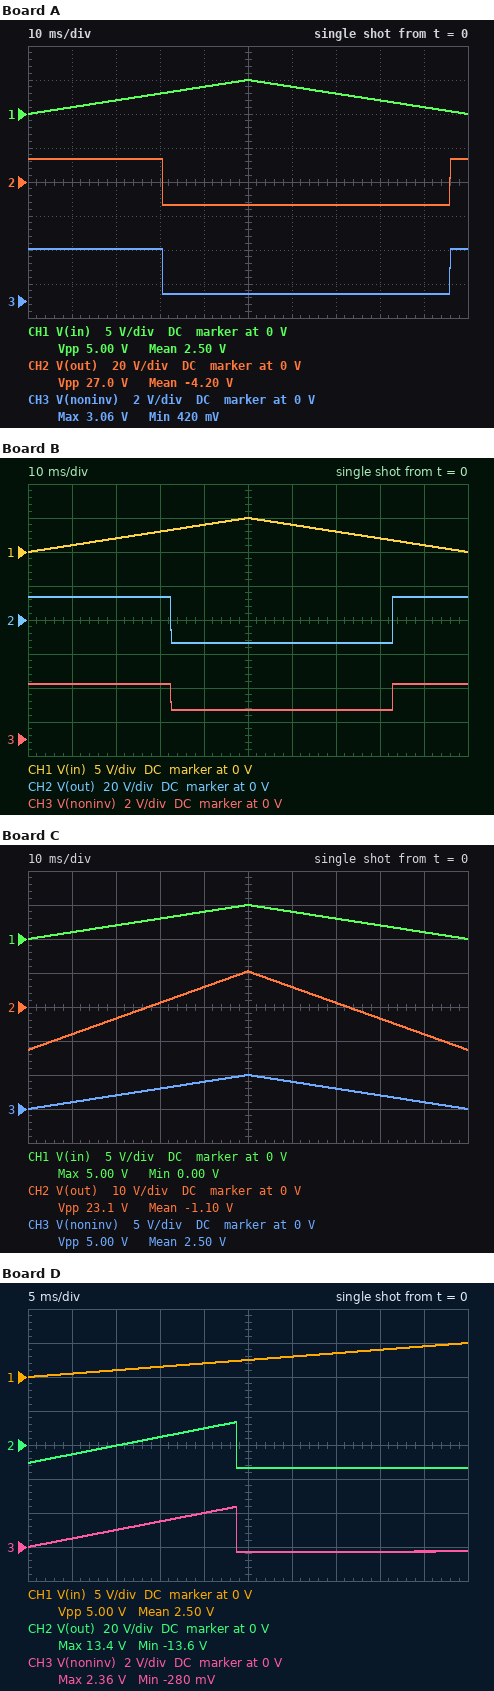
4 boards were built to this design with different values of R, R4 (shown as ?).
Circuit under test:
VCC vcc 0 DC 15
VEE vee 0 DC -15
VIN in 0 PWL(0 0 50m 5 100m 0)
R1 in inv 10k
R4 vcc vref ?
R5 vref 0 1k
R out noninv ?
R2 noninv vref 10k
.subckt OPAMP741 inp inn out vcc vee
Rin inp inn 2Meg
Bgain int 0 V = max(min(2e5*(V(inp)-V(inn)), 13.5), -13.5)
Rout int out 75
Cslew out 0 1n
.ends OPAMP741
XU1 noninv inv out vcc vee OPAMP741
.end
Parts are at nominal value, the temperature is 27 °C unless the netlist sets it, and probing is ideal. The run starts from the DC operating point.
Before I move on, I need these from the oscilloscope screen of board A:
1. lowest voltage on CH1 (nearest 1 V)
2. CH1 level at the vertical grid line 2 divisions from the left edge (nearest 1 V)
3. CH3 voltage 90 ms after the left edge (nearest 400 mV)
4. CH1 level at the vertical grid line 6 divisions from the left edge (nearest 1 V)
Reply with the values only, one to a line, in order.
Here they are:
0 V
2 V
400 mV
4 V
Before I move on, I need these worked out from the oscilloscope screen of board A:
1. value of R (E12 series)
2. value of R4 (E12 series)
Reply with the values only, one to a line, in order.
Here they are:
100 kΩ
6.8 kΩ
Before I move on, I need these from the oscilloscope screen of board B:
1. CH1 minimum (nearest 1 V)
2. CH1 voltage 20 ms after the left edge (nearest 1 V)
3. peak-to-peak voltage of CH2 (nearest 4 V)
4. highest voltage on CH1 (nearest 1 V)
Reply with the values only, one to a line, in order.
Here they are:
0 V
2 V
28 V
5 V
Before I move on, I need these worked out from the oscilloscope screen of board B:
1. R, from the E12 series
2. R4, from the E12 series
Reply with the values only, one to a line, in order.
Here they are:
180 kΩ
4.7 kΩ
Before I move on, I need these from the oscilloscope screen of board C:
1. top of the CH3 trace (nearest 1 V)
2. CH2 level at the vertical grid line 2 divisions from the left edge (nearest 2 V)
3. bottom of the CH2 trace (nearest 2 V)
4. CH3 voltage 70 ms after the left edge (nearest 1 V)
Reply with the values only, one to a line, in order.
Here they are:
5 V
-4 V
-12 V
3 V
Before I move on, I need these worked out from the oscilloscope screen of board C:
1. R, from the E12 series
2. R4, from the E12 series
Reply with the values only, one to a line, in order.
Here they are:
39 kΩ
3.3 kΩ
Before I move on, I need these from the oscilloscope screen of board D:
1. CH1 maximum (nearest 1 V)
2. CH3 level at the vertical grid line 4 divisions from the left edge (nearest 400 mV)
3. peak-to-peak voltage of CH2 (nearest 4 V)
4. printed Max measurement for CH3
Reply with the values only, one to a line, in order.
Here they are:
5 V
2.0 V
28 V
2.36 V
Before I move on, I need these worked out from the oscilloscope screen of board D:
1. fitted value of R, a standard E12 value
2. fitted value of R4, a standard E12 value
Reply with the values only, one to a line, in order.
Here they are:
100 kΩ
12 kΩ
